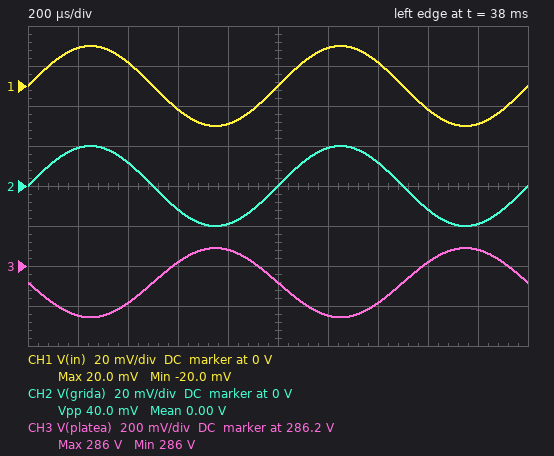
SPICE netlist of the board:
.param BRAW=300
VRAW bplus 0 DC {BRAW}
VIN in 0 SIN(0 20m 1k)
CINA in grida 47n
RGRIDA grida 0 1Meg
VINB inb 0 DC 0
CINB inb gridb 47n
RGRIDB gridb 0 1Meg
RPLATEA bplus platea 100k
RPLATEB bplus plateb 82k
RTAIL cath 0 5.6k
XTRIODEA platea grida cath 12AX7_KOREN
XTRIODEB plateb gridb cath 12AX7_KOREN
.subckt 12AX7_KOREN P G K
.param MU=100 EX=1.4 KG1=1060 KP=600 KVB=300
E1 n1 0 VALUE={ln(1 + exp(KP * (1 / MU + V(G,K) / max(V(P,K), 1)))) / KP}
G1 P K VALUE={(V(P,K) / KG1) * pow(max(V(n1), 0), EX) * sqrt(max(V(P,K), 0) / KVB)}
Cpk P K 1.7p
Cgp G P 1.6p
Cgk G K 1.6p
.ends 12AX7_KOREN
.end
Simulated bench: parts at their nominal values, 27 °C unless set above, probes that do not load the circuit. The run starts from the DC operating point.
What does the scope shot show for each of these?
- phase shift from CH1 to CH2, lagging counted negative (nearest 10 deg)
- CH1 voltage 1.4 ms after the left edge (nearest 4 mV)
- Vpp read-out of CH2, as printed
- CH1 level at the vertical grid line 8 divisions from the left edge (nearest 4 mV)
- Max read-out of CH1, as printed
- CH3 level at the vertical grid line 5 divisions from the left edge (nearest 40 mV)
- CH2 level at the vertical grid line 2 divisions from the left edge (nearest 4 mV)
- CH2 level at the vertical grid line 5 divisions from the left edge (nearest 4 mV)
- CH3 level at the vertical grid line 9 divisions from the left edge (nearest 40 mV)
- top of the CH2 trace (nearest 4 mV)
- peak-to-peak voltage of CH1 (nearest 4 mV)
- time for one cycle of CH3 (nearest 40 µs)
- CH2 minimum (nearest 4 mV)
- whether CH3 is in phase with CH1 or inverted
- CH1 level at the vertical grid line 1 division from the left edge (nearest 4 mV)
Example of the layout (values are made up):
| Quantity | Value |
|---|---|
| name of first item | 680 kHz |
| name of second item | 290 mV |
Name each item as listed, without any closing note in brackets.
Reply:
| Quantity | Value |
|---|---|
| phase shift from CH1 to CH2, lagging counted negative | 0 deg |
| CH1 voltage 1.4 ms after the left edge | 12 mV |
| Vpp read-out of CH2, as printed | 40.0 mV |
| CH1 level at the vertical grid line 8 divisions from the left edge | -12 mV |
| Max read-out of CH1, as printed | 20.0 mV |
| CH3 level at the vertical grid line 5 divisions from the left edge | 286.12 V |
| CH2 level at the vertical grid line 2 divisions from the left edge | 12 mV |
| CH2 level at the vertical grid line 5 divisions from the left edge | 0 V |
| CH3 level at the vertical grid line 9 divisions from the left edge | 286.28 V |
| top of the CH2 trace | 20 mV |
| peak-to-peak voltage of CH1 | 40 mV |
| time for one cycle of CH3 | 1.00 ms |
| CH2 minimum | -20 mV |
| whether CH3 is in phase with CH1 or inverted | inverted |
| CH1 level at the vertical grid line 1 division from the left edge | 20 mV |
